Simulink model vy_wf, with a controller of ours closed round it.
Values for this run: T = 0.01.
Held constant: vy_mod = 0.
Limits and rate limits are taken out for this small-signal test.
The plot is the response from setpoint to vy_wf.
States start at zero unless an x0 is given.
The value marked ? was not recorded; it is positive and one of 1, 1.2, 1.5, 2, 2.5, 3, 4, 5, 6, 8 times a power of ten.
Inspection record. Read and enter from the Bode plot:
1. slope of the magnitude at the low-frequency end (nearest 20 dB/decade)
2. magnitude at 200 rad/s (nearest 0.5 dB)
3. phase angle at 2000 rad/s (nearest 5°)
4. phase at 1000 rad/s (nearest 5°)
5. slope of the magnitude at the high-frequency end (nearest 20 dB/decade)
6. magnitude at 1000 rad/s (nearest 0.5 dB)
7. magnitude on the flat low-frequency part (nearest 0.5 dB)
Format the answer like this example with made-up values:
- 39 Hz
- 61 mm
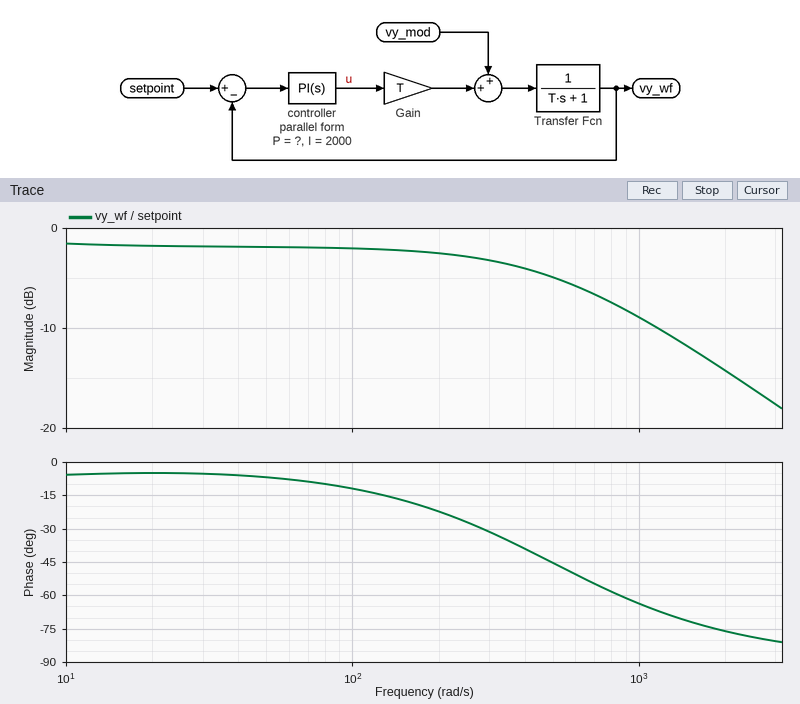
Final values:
- 0 dB/decade
- -2.5 dB
- -75°
- -65°
- -20 dB/decade
- -9.0 dB
- -1.5 dB
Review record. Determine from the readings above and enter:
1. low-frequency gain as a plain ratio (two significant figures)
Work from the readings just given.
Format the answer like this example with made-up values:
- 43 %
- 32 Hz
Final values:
- 0.84
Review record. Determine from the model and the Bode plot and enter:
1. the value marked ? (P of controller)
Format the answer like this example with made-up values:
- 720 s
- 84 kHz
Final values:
- 400
